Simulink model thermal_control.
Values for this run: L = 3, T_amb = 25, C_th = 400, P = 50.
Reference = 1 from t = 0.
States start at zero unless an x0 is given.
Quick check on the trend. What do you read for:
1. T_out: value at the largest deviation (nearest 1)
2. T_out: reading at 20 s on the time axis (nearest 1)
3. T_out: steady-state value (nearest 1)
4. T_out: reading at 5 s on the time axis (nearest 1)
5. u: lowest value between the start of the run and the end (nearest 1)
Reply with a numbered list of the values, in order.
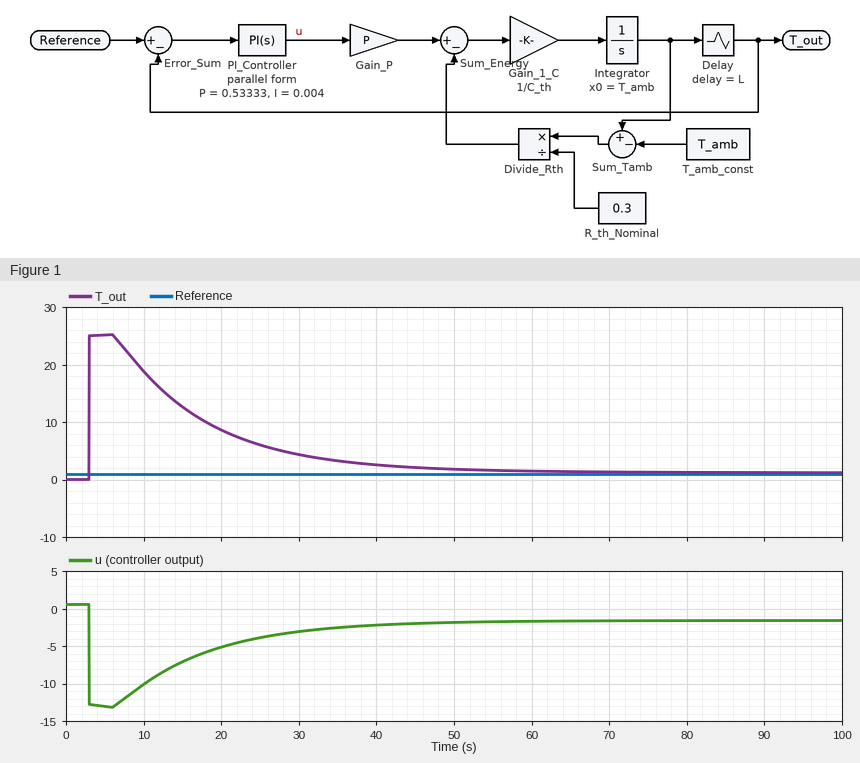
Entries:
1. 25
2. 9
3. 1
4. 25
5. -13
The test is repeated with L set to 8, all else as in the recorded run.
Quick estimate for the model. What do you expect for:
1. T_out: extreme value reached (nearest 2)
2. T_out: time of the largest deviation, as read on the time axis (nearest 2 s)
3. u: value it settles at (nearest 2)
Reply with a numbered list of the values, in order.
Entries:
1. 26
2. 16 s
3. -2
